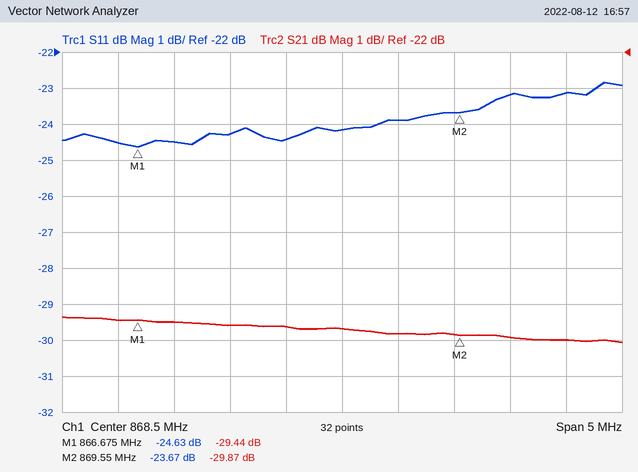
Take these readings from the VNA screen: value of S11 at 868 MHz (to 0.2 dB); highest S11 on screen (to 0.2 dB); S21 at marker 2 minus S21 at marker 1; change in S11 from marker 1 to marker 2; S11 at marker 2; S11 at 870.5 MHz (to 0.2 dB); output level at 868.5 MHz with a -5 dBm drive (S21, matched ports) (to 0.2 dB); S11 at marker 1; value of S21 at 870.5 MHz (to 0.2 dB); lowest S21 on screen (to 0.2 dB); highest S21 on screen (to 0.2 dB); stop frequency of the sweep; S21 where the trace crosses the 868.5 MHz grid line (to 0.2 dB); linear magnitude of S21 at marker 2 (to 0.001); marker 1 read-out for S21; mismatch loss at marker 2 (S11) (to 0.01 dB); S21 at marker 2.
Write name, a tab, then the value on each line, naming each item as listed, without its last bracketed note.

value of S11 at 868 MHz	-24.4 dB
highest S11 on screen	-22.8 dB
S21 at marker 2 minus S21 at marker 1	-0.43 dB
change in S11 from marker 1 to marker 2	0.96 dB
S11 at marker 2	-23.67 dB
S11 at 870.5 MHz	-23.2 dB
output level at 868.5 MHz with a -5 dBm drive (S21, matched ports)	-34.6 dBm
S11 at marker 1	-24.63 dB
value of S21 at 870.5 MHz	-30.0 dB
lowest S21 on screen	-30.0 dB
highest S21 on screen	-29.4 dB
stop frequency of the sweep	871 MHz
S21 where the trace crosses the 868.5 MHz grid line	-29.6 dB
linear magnitude of S21 at marker 2	0.032
marker 1 read-out for S21	-29.44 dB
mismatch loss at marker 2 (S11)	0.02 dB
S21 at marker 2	-29.87 dB
